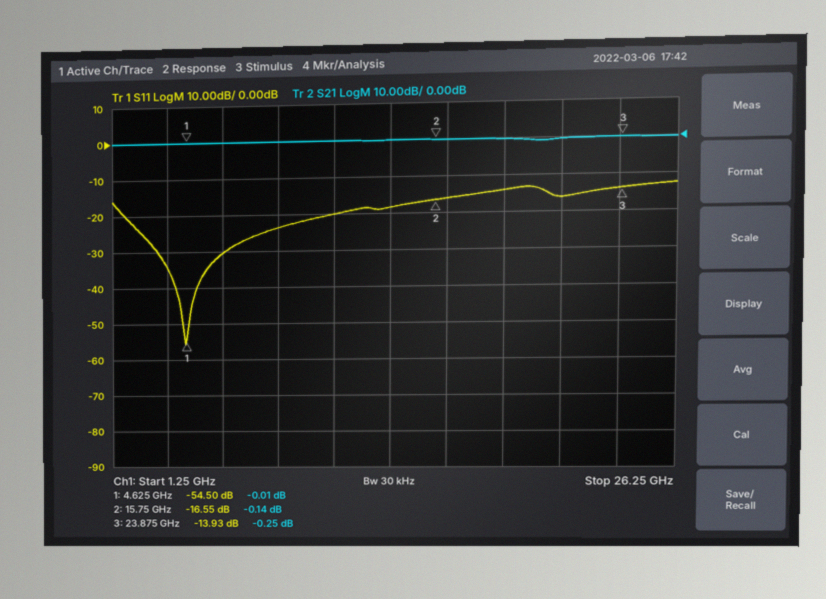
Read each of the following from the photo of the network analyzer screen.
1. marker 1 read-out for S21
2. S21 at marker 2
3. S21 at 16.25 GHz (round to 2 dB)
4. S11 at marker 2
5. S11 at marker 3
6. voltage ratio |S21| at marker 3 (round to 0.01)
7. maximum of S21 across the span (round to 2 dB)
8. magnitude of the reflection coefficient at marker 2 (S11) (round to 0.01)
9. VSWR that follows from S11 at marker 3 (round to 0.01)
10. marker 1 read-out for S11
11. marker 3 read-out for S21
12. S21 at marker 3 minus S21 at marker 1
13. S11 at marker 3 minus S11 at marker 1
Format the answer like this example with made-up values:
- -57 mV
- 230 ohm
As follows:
- -0.01 dB
- -0.14 dB
- 0 dB
- -16.55 dB
- -13.93 dB
- 0.97
- 0 dB
- 0.15
- 1.50
- -54.50 dB
- -0.25 dB
- -0.24 dB
- 40.57 dB
